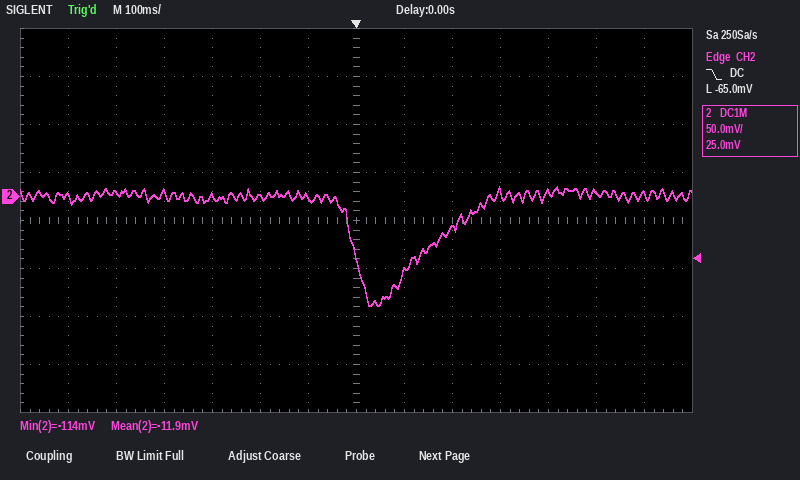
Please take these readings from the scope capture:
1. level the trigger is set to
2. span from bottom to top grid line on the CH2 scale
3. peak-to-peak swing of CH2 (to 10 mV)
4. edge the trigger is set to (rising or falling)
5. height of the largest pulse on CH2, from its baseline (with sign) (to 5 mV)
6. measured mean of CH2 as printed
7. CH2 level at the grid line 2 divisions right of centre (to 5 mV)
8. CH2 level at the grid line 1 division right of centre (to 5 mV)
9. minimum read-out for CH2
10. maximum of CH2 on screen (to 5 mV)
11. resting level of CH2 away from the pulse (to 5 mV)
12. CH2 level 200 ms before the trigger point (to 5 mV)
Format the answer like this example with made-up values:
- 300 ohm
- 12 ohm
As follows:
- -65.0 mV
- 400 mV
- 120 mV
- falling
- -115 mV
- -11.9 mV
- -30 mV
- -80 mV
- -114 mV
- 10 mV
- 0 mV
- 0 mV
